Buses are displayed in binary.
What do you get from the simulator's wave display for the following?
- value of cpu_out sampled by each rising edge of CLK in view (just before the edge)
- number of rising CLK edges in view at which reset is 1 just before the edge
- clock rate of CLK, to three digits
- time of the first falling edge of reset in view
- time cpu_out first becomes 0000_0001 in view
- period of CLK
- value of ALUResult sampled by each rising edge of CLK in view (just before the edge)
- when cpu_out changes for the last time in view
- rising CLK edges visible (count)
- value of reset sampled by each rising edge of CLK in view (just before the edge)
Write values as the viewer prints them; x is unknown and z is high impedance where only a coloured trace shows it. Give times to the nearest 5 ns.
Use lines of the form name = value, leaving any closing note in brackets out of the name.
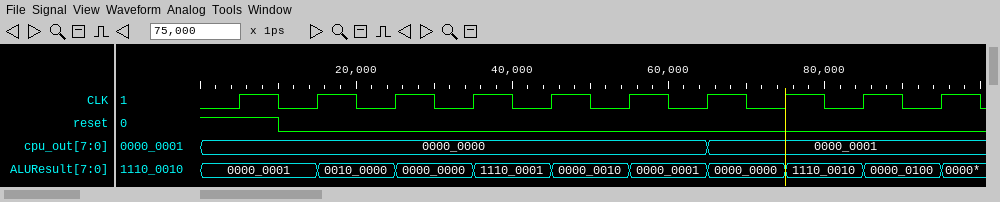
value of cpu_out sampled by each rising edge of CLK in view = 0000_0000, 0000_0000, 0000_0000, 0000_0000, 0000_0000, 0000_0000, 0000_0000, 0000_0001, 0000_0001, 0000_0001
number of rising CLK edges in view at which reset is 1 just before the edge = 1
clock rate of CLK, to three digits = 100 MHz
time of the first falling edge of reset in view = 10 ns
time cpu_out first becomes 0000_0001 in view = 65 ns
period of CLK = 10 ns
value of ALUResult sampled by each rising edge of CLK in view = 0000_0001, 0000_0001, 0010_0000, 0000_0000, 1110_0001, 0000_0010, 0000_0001, 0000_0000, 1110_0010, 0000_0100
when cpu_out changes for the last time in view = 65 ns
rising CLK edges visible = 10
value of reset sampled by each rising edge of CLK in view = 1 0 0 0 0 0 0 0 0 0
